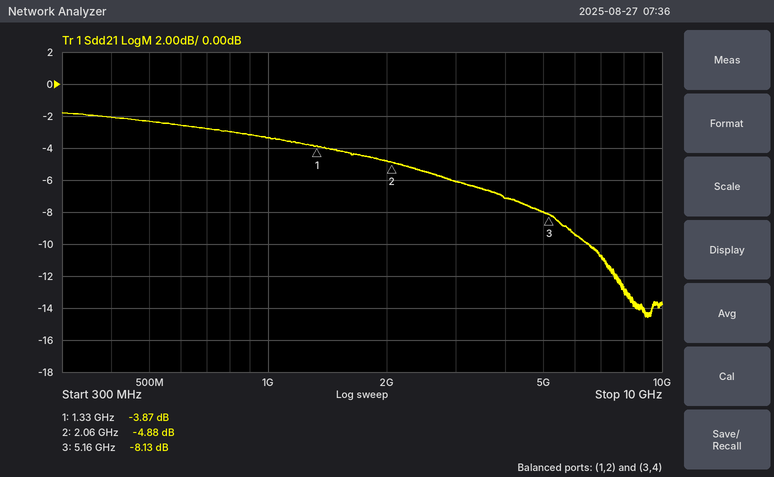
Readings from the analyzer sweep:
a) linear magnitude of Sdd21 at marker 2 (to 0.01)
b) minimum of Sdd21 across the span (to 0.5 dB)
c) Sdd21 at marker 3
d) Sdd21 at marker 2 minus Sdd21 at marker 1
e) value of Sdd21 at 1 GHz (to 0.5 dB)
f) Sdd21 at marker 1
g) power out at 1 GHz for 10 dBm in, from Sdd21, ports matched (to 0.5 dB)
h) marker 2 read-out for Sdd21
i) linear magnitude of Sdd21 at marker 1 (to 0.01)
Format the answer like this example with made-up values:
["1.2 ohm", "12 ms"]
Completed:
["0.57", "-14.5 dB", "-8.13 dB", "-1.01 dB", "-3.5 dB", "-3.87 dB", "6.5 dBm", "-4.88 dB", "0.64"]
